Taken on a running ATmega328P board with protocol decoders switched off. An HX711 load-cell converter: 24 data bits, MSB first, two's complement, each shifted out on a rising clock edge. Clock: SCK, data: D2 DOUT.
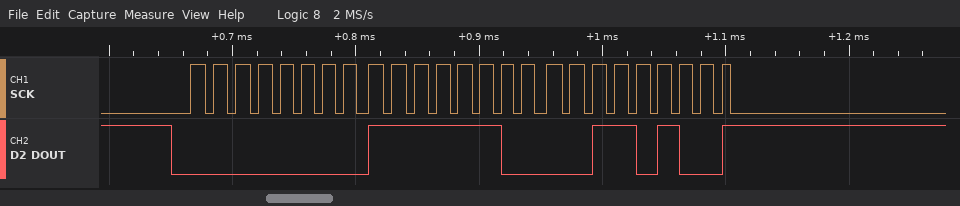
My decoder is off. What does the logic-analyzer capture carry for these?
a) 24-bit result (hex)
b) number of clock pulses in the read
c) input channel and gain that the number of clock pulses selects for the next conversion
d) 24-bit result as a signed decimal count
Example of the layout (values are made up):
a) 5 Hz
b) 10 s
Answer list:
a) 0x00FC34
b) 25
c) channel A, gain 128
d) 64564
